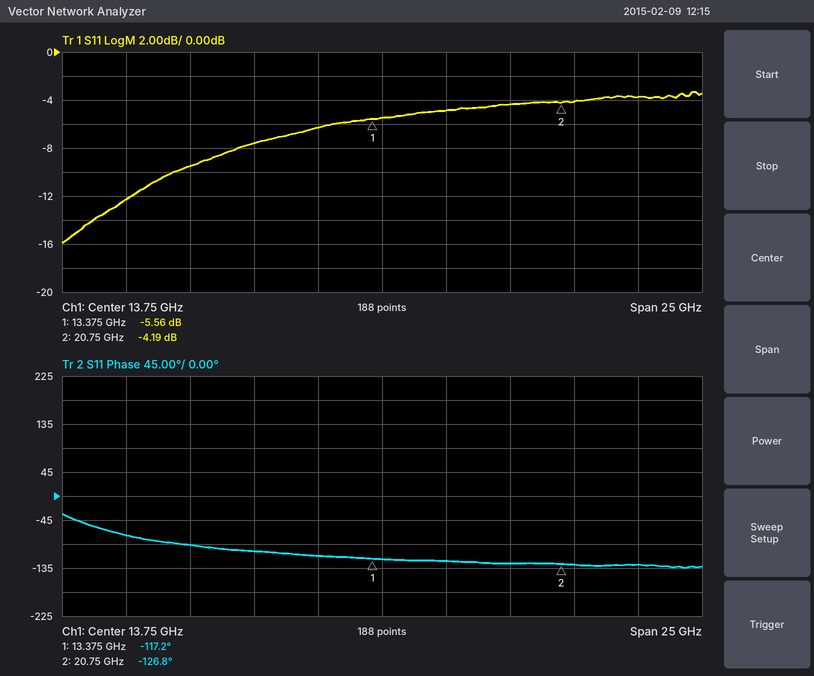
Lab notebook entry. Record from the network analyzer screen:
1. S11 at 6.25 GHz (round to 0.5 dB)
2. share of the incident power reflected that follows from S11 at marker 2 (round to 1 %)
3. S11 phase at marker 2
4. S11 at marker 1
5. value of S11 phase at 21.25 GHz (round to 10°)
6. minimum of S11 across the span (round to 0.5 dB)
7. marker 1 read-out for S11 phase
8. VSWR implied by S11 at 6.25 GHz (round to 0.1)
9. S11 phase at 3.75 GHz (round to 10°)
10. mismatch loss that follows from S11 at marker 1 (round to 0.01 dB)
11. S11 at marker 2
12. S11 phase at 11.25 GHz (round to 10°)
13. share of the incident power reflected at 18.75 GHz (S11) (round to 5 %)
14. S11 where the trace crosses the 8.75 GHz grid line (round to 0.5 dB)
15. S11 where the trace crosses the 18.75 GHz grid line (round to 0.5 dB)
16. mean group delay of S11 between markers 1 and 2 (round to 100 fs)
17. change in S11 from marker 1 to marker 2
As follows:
-9.5 dB
38 %
-126.8°
-5.56 dB
-130°
-16.0 dB
-117.2°
2.0
-70°
1.41 dB
-4.19 dB
-110°
35 %
-7.5 dB
-4.5 dB
3.6 ps
1.37 dB
